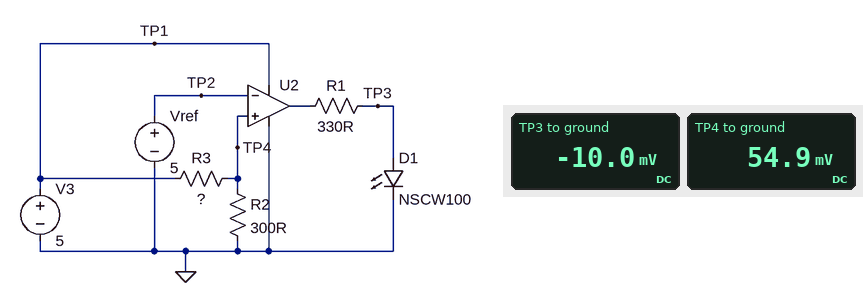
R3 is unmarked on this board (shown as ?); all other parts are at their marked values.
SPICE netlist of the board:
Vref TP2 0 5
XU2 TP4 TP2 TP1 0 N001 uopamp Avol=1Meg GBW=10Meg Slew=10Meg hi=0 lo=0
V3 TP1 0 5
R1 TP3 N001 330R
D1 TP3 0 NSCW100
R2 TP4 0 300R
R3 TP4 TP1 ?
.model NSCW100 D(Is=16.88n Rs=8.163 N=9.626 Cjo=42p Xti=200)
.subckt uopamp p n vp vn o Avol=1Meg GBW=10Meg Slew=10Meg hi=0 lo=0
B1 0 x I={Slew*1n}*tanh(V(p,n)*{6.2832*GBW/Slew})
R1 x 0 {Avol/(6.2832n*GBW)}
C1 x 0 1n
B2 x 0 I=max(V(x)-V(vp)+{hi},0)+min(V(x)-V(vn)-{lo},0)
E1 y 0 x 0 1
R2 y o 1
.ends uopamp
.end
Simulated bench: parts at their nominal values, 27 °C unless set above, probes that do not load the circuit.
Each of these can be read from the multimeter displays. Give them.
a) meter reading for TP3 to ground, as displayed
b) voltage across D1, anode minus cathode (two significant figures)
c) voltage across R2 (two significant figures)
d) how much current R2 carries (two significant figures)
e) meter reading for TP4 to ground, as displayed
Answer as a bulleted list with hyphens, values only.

- -10.0 mV
- -10 mV
- 55 mV
- 180 µA
- 54.9 mV
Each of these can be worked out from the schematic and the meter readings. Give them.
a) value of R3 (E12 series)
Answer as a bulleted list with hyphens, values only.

- 27 kΩ
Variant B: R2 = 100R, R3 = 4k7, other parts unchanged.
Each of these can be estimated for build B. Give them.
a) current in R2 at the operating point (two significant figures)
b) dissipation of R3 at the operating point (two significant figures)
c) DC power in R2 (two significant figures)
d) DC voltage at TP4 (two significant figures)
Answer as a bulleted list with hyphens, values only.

- 1.0 mA
- 5.1 mW
- 110 µW
- 100 mV
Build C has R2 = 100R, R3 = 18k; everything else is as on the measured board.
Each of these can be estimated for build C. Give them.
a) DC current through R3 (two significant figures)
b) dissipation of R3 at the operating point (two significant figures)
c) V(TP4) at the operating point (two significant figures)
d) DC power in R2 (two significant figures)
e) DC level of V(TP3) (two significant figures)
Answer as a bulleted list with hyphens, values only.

- 280 µA
- 1.4 mW
- 28 mV
- 7.6 µW
- -10 mV
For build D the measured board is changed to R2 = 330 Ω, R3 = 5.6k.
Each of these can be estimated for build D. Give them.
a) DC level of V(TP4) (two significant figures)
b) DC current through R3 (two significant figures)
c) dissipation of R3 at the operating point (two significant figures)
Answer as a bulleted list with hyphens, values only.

- 280 mV
- 840 µA
- 4.0 mW
